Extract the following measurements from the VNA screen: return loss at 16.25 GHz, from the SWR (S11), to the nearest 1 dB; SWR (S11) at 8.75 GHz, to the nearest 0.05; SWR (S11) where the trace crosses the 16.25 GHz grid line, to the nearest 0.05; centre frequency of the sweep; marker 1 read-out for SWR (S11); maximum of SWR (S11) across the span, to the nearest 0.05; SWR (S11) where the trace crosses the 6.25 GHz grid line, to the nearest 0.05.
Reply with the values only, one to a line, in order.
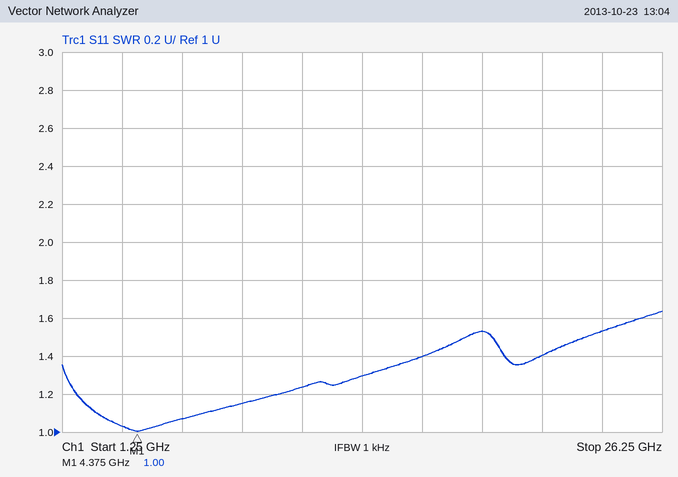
16 dB
1.15
1.40
13.75 GHz
1.00
1.65
1.05
